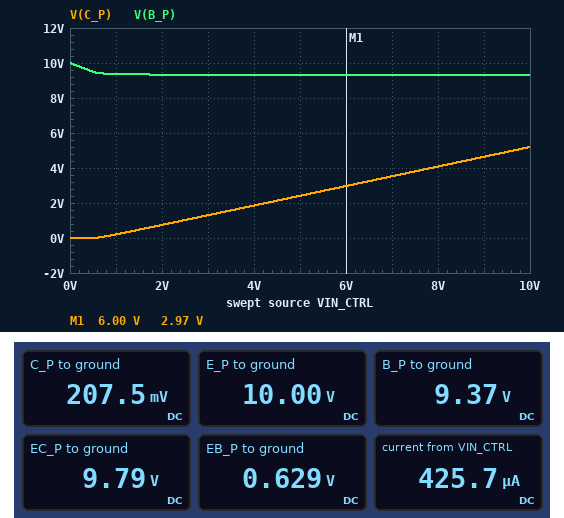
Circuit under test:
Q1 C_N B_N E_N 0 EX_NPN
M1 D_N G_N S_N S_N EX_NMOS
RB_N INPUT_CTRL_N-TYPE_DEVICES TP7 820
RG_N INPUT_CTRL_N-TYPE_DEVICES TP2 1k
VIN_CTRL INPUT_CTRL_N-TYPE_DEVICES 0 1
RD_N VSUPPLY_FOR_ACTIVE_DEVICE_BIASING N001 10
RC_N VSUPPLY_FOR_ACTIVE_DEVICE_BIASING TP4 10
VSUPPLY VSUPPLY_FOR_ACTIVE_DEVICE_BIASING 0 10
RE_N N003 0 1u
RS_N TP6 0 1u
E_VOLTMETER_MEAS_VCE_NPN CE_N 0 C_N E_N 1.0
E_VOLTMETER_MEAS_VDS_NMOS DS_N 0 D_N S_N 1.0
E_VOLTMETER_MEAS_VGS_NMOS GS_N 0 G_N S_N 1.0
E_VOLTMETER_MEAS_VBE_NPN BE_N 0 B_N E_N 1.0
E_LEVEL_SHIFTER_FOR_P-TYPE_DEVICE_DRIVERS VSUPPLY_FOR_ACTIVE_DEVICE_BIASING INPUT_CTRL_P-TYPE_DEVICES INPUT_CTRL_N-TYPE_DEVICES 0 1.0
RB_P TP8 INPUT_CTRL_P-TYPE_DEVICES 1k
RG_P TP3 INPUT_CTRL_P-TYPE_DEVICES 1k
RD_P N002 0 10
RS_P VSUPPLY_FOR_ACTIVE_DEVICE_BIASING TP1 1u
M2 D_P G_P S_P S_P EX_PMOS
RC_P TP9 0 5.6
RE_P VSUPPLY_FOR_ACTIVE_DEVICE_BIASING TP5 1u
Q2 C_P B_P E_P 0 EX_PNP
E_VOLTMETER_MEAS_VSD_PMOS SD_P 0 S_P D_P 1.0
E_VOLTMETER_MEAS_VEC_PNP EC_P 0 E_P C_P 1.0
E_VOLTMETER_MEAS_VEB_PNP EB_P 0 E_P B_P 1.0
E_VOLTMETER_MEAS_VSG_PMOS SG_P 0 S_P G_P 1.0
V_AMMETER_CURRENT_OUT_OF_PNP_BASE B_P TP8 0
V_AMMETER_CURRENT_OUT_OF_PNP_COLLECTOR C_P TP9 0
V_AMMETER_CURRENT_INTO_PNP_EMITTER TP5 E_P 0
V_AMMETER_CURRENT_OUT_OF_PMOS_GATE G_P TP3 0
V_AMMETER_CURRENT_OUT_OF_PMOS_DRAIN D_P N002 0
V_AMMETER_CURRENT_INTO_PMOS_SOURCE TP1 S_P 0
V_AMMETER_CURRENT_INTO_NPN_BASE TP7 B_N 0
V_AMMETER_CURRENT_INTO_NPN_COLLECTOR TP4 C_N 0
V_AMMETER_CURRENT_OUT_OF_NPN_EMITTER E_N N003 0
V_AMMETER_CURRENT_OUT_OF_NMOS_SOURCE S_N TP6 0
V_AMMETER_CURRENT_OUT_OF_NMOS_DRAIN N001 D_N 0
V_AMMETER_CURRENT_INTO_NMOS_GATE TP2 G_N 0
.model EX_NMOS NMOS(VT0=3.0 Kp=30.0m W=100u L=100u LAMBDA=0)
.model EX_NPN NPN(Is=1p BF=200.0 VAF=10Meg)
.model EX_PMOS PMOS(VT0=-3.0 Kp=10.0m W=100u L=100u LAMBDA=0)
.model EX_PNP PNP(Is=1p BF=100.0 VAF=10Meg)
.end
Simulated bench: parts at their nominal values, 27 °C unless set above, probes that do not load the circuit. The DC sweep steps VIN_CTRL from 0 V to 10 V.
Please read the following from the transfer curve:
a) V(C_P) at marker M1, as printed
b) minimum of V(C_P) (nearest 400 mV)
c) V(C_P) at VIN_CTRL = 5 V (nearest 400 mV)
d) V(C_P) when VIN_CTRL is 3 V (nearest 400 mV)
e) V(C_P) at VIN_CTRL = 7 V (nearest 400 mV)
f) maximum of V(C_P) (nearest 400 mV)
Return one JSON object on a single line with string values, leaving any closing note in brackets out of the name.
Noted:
{"V(C_P) at marker M1, as printed": "2.97 V", "minimum of V(C_P)": "0 V", "V(C_P) at VIN_CTRL = 5 V": "2.4 V", "V(C_P) when VIN_CTRL is 3 V": "1.2 V", "V(C_P) at VIN_CTRL = 7 V": "3.6 V", "maximum of V(C_P)": "5.2 V"}
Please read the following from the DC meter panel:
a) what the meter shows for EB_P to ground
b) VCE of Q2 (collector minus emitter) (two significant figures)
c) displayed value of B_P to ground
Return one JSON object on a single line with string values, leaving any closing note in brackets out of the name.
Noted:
{"what the meter shows for EB_P to ground": "0.629 V", "VCE of Q2 (collector minus emitter)": "-9.8 V", "displayed value of B_P to ground": "9.37 V"}
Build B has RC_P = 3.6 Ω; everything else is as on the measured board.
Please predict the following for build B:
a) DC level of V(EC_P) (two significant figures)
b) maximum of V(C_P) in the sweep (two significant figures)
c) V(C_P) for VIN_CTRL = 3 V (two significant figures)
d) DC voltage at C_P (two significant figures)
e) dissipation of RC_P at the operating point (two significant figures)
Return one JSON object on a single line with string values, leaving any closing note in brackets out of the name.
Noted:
{"DC level of V(EC_P)": "9.9 V", "maximum of V(C_P) in the sweep": "3.3 V", "V(C_P) for VIN_CTRL = 3 V": "840 mV", "DC voltage at C_P": "130 mV", "dissipation of RC_P at the operating point": "4.9 mW"}
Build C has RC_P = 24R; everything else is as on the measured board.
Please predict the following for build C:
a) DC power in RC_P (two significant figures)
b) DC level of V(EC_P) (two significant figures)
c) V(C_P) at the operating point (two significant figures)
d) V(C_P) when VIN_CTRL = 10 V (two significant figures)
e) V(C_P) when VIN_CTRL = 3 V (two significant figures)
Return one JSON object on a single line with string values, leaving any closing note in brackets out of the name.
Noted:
{"DC power in RC_P": "33 mW", "DC level of V(EC_P)": "9.1 V", "V(C_P) at the operating point": "890 mV", "V(C_P) when VIN_CTRL = 10 V": "9.9 V", "V(C_P) when VIN_CTRL = 3 V": "5.6 V"}
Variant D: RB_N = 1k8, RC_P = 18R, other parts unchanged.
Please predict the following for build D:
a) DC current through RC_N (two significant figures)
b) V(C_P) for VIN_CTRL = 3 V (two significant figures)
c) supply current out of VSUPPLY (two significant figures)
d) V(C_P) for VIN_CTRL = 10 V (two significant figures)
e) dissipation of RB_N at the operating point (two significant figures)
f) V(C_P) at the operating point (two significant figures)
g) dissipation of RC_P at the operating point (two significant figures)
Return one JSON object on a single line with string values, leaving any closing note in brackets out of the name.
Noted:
{"DC current through RC_N": "41 mA", "V(C_P) for VIN_CTRL = 3 V": "4.2 V", "supply current out of VSUPPLY": "78 mA", "V(C_P) for VIN_CTRL = 10 V": "9.9 V", "dissipation of RB_N at the operating point": "75 µW", "V(C_P) at the operating point": "670 mV", "dissipation of RC_P at the operating point": "25 mW"}
